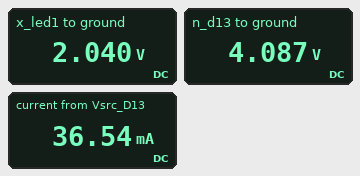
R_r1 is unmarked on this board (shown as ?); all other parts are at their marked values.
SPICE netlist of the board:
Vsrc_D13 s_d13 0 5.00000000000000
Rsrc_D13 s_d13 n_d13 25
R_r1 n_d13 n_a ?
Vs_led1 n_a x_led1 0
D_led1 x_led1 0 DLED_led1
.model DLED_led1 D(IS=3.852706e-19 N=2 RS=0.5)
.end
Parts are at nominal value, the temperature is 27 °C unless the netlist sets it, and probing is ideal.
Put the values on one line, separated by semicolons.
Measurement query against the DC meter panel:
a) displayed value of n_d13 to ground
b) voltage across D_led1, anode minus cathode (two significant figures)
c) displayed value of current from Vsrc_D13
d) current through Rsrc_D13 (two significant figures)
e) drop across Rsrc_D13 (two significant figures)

4.087 V; 2.0 V; 36.54 mA; 37 mA; 910 mV
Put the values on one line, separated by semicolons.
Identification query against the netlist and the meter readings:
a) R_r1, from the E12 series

56 Ω
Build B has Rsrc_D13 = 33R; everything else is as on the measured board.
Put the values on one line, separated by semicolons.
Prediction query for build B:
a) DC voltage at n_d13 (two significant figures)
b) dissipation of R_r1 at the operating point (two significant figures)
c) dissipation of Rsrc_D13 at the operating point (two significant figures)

3.9 V; 62 mW; 37 mW
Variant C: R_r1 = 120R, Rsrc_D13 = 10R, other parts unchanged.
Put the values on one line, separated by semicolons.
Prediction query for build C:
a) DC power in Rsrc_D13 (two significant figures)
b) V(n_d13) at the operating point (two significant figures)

5.3 mW; 4.8 V
